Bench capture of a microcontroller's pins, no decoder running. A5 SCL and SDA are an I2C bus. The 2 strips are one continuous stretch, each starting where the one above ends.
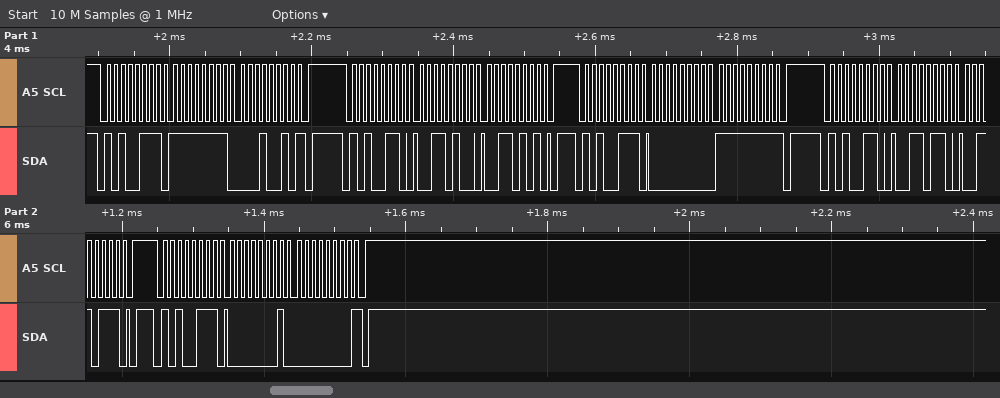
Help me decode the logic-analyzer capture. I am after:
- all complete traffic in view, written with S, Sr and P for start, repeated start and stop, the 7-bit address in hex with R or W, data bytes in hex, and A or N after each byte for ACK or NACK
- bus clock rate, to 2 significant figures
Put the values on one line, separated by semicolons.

S 53R A FF A 12 N P S 53W A 34 A 35 A P S 53R A 00 A FF N P S 53W A 36 A 37 A P S 53R A 01 A 00 N P; 100 kHz
